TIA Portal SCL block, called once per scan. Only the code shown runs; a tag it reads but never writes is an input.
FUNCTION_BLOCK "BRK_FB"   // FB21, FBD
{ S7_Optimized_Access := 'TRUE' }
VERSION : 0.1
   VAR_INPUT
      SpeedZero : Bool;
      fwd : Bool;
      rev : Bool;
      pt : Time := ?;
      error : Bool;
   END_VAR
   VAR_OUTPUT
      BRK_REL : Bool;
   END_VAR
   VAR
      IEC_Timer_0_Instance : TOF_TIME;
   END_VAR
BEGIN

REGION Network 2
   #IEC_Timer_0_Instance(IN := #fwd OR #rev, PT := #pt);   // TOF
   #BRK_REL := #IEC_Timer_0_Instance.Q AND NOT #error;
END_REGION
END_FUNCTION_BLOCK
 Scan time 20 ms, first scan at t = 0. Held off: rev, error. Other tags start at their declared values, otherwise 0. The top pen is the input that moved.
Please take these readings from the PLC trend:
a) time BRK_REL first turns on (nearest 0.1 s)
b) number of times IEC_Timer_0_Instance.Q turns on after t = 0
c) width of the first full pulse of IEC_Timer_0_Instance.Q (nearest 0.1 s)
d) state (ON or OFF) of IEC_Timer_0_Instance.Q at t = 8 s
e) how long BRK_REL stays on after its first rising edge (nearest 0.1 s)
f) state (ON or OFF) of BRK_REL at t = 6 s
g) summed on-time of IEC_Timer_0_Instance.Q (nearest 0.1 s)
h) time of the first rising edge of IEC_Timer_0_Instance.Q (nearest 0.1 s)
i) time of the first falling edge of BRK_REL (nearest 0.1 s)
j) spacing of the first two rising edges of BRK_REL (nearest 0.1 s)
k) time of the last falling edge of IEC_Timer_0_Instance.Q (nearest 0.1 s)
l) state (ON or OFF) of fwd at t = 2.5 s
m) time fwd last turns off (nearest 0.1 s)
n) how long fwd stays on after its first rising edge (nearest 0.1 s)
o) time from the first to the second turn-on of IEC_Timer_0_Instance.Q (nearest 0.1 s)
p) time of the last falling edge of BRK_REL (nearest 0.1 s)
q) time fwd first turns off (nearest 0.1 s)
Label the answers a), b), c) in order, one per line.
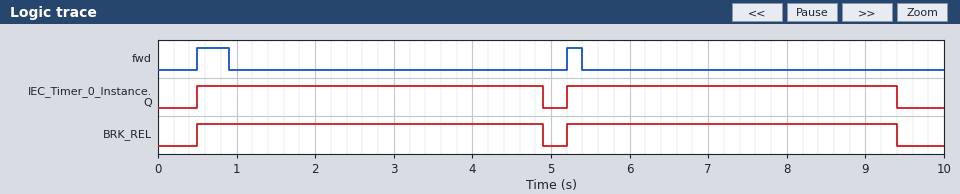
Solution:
a) 0.5 s
b) 2
c) 4.4 s
d) ON
e) 4.4 s
f) ON
g) 8.6 s
h) 0.5 s
i) 4.9 s
j) 4.7 s
k) 9.4 s
l) OFF
m) 5.4 s
n) 0.4 s
o) 4.7 s
p) 9.4 s
q) 0.9 s
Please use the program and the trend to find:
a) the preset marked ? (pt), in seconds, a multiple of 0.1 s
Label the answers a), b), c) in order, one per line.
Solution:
a) 4.0 s
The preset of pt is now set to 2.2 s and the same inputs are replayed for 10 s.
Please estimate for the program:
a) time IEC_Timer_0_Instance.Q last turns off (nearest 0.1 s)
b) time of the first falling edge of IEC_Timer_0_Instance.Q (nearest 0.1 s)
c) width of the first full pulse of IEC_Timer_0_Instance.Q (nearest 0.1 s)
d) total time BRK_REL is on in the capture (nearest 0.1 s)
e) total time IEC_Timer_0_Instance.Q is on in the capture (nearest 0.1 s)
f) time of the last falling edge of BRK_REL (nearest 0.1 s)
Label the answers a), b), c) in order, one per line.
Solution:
a) 7.6 s
b) 3.1 s
c) 2.6 s
d) 5.0 s
e) 5.0 s
f) 7.6 s
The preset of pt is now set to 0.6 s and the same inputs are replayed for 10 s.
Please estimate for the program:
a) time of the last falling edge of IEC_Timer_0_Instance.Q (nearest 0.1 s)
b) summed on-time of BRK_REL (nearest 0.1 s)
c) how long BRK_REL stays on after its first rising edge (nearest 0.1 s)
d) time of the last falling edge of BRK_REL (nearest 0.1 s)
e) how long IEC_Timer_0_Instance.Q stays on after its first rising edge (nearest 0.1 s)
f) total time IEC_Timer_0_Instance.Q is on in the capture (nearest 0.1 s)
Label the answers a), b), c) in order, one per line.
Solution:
a) 6.0 s
b) 1.8 s
c) 1.0 s
d) 6.0 s
e) 1.0 s
f) 1.8 s
